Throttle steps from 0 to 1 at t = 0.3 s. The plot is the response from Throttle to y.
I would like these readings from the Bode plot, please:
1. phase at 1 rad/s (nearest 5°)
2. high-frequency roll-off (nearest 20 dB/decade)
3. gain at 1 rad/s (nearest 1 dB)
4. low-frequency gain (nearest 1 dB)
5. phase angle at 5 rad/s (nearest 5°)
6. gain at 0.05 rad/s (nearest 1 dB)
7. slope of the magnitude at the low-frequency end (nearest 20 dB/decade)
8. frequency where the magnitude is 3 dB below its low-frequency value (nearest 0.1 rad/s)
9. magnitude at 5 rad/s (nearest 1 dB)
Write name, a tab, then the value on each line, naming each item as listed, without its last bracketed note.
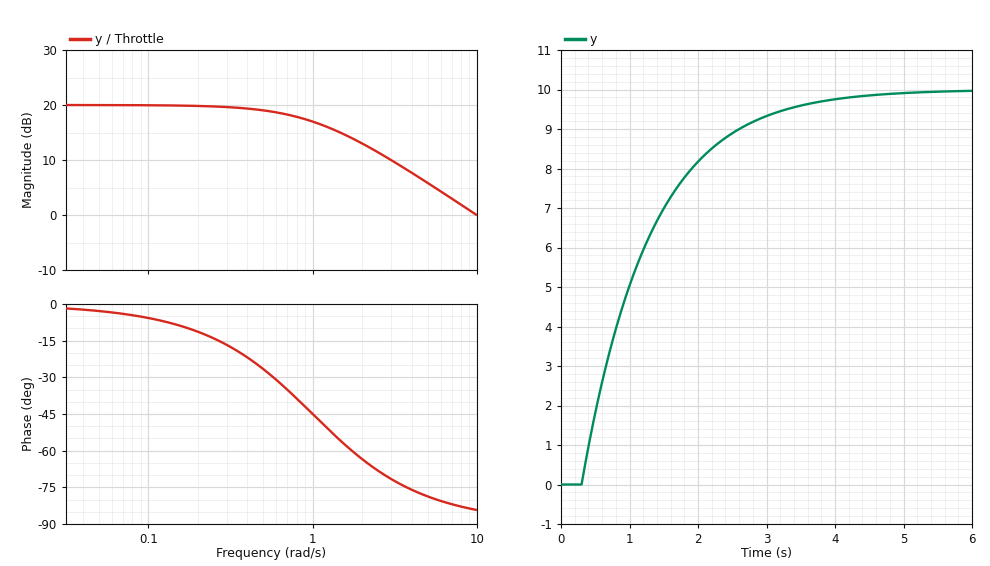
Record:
phase at 1 rad/s	-45°
high-frequency roll-off	-20 dB/decade
gain at 1 rad/s	17 dB
low-frequency gain	20 dB
phase angle at 5 rad/s	-80°
gain at 0.05 rad/s	20 dB
slope of the magnitude at the low-frequency end	0 dB/decade
frequency where the magnitude is 3 dB below its low-frequency value	1.0 rad/s
magnitude at 5 rad/s	6 dB
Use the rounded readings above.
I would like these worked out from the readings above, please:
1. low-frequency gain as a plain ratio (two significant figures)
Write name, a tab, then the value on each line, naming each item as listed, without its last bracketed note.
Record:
low-frequency gain as a plain ratio	10
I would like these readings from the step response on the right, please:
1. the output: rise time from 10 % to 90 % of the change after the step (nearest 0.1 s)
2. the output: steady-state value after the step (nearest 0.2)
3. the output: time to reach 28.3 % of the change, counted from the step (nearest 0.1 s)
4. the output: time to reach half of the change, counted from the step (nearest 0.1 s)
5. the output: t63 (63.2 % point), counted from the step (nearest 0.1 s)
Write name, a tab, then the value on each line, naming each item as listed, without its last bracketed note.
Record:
the output: rise time from 10 % to 90 % of the change after the step	2.2 s
the output: steady-state value after the step	10.0
the output: time to reach 28.3 % of the change, counted from the step	0.3 s
the output: time to reach half of the change, counted from the step	0.7 s
the output: t63 (63.2 % point), counted from the step	1.0 s
